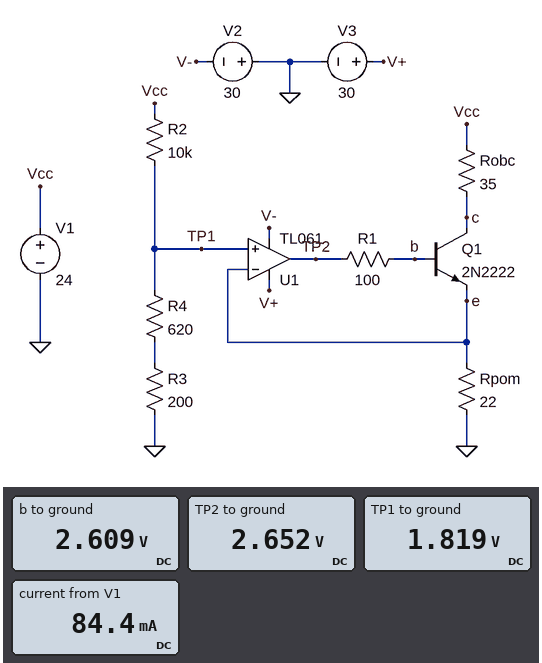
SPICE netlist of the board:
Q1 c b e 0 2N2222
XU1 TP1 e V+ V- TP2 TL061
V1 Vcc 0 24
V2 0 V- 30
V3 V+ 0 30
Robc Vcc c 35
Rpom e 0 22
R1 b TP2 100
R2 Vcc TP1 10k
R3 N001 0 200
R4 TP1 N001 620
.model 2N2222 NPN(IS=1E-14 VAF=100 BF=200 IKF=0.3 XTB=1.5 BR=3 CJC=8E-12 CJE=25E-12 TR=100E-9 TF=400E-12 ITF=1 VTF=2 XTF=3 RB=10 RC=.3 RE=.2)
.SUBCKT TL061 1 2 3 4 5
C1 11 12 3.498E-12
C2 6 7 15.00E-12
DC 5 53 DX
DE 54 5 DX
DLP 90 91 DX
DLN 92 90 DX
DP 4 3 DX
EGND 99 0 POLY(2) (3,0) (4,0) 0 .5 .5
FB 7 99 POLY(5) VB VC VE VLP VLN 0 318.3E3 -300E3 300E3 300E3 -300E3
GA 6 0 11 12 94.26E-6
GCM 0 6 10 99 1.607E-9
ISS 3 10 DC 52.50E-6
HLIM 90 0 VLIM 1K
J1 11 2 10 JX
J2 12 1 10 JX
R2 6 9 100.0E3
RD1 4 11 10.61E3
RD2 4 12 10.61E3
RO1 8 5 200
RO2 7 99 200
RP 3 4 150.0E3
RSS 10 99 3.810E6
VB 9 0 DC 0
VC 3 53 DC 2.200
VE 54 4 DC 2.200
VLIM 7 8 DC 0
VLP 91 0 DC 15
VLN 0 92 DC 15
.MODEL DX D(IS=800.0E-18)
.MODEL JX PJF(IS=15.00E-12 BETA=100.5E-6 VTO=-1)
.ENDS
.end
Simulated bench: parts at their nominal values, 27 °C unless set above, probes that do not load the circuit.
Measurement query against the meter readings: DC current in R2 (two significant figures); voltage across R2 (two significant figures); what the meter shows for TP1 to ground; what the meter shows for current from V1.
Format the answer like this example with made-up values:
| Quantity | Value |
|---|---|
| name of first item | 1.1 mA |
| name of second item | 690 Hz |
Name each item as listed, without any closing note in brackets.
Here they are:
| Quantity | Value |
|---|---|
| DC current in R2 | 2.2 mA |
| voltage across R2 | 22 V |
| what the meter shows for TP1 to ground | 1.819 V |
| what the meter shows for current from V1 | 84.4 mA |
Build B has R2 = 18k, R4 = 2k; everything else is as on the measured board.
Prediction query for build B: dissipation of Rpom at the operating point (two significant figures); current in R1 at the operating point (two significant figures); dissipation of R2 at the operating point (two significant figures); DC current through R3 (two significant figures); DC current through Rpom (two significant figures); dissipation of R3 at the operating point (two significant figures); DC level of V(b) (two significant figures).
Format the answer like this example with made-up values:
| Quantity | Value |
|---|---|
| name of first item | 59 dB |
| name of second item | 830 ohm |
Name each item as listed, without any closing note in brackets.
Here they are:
| Quantity | Value |
|---|---|
| dissipation of Rpom at the operating point | 310 mW |
| current in R1 at the operating point | 680 µA |
| dissipation of R2 at the operating point | 25 mW |
| DC current through R3 | 1.2 mA |
| DC current through Rpom | 120 mA |
| dissipation of R3 at the operating point | 280 µW |
| DC level of V(b) | 3.4 V |
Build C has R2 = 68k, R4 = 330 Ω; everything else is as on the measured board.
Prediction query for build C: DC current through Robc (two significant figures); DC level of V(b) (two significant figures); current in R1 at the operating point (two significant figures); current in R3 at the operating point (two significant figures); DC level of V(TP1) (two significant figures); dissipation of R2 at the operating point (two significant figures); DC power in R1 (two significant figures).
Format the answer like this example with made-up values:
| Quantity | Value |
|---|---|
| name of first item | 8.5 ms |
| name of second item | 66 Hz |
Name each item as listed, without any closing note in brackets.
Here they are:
| Quantity | Value |
|---|---|
| DC current through Robc | 8.4 mA |
| DC level of V(b) | 890 mV |
| current in R1 at the operating point | 35 µA |
| current in R3 at the operating point | 350 µA |
| DC level of V(TP1) | 190 mV |
| dissipation of R2 at the operating point | 8.3 mW |
| DC power in R1 | 120 nW |
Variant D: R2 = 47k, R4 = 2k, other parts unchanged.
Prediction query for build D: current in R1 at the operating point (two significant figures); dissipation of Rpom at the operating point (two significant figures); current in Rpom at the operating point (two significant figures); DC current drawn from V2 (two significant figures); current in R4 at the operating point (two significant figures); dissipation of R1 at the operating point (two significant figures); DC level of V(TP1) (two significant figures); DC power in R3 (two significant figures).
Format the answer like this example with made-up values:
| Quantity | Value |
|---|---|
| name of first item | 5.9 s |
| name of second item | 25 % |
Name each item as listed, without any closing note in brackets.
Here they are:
| Quantity | Value |
|---|---|
| current in R1 at the operating point | 230 µA |
| dissipation of Rpom at the operating point | 52 mW |
| current in Rpom at the operating point | 49 mA |
| DC current drawn from V2 | 450 µA |
| current in R4 at the operating point | 490 µA |
| dissipation of R1 at the operating point | 5.2 µW |
| DC level of V(TP1) | 1.1 V |
| DC power in R3 | 48 µW |
